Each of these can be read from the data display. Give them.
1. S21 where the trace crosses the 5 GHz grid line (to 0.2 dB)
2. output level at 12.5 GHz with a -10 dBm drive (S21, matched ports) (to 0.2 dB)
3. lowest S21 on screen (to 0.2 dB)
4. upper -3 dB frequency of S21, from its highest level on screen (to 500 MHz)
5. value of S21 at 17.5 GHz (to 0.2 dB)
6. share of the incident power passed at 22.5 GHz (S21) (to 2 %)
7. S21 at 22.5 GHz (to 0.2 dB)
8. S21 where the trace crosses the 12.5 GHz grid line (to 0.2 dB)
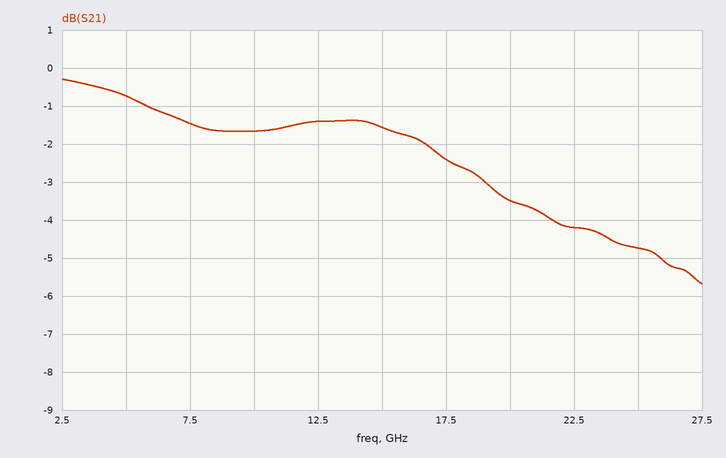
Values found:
-0.8 dB
-11.4 dBm
-5.6 dB
19.5 GHz
-2.4 dB
38 %
-4.2 dB
-1.4 dB
